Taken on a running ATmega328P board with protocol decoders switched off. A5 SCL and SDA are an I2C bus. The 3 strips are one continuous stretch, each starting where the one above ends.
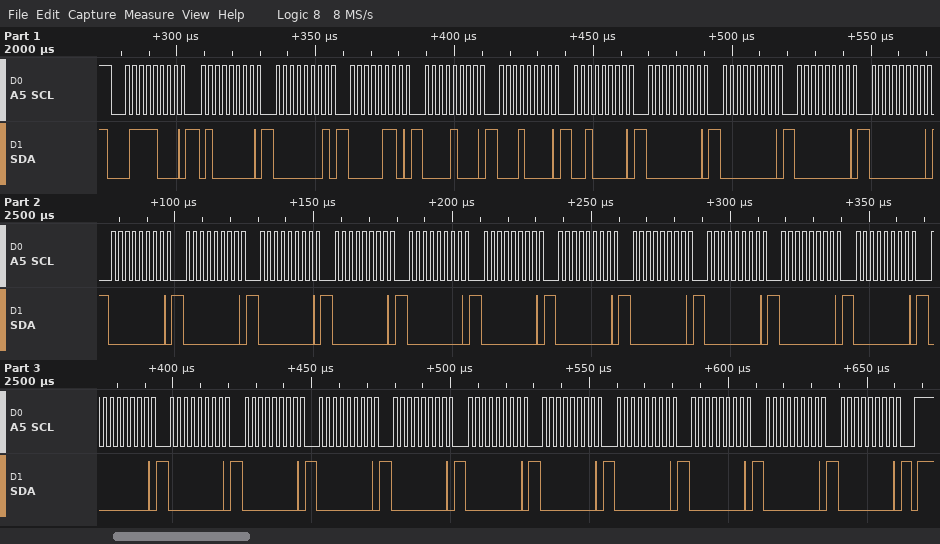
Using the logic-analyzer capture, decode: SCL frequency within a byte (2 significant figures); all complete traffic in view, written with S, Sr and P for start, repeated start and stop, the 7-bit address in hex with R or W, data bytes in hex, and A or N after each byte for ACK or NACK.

400 kHz
S 3CW A 40 A 01 A 06 A 08 A 10 A 20 A 00 A 00 A 00 A 00 A 00 A 00 A 00 A 00 A 00 A 00 A 00 A 00 A 00 A 00 A 00 A 00 A 00 A 00 A 00 A 00 A 00 A 00 A 00 A 00 A 00 A 00 A P
